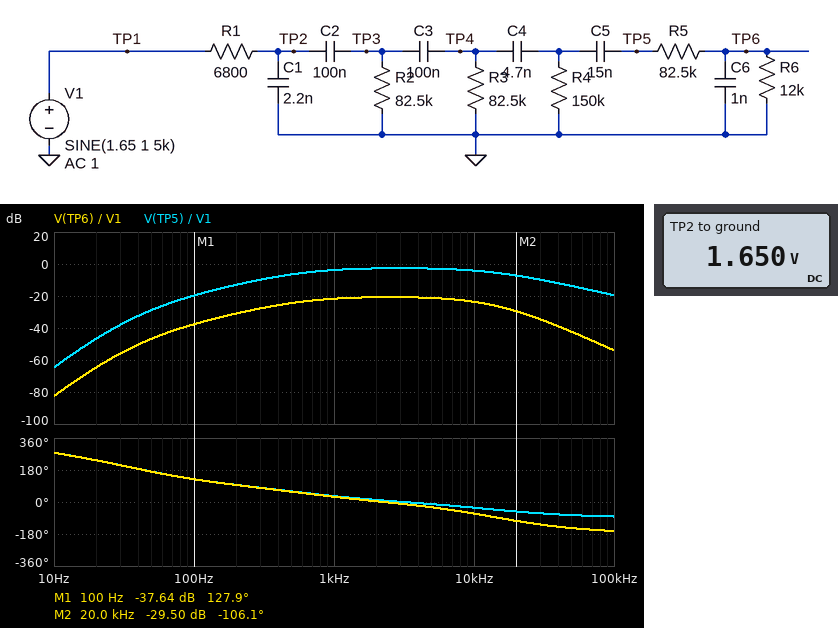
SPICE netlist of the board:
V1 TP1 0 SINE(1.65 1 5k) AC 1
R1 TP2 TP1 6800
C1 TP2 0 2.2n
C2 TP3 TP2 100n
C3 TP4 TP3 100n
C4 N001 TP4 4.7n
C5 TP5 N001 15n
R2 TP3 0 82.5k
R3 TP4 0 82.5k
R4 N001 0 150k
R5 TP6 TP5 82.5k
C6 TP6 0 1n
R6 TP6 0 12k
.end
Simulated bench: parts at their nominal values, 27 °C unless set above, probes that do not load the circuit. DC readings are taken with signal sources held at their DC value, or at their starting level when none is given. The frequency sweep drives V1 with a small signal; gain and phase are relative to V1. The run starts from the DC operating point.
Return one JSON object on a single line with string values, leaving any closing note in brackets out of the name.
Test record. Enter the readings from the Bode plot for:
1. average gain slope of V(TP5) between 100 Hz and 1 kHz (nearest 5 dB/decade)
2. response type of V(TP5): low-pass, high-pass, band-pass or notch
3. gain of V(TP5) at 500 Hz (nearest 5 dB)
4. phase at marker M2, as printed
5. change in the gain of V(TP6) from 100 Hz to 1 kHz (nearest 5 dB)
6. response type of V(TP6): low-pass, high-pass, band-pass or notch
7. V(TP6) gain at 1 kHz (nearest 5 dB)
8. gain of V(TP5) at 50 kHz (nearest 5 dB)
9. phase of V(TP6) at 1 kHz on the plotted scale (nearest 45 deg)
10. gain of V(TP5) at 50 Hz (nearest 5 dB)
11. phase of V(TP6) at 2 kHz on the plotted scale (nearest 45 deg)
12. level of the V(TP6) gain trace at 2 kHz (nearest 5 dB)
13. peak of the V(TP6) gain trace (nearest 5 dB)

{"average gain slope of V(TP5) between 100 Hz and 1 kHz": "15 dB/decade", "response type of V(TP5): low-pass, high-pass, band-pass or notch": "band-pass", "gain of V(TP5) at 500 Hz": "-5 dB", "phase at marker M2, as printed": "-106.1 deg", "change in the gain of V(TP6) from 100 Hz to 1 kHz": "15 dB", "response type of V(TP6): low-pass, high-pass, band-pass or notch": "band-pass", "V(TP6) gain at 1 kHz": "-20 dB", "gain of V(TP5) at 50 kHz": "-15 dB", "phase of V(TP6) at 1 kHz on the plotted scale": "45 deg", "gain of V(TP5) at 50 Hz": "-30 dB", "phase of V(TP6) at 2 kHz on the plotted scale": "0 deg", "level of the V(TP6) gain trace at 2 kHz": "-20 dB", "peak of the V(TP6) gain trace": "-20 dB"}
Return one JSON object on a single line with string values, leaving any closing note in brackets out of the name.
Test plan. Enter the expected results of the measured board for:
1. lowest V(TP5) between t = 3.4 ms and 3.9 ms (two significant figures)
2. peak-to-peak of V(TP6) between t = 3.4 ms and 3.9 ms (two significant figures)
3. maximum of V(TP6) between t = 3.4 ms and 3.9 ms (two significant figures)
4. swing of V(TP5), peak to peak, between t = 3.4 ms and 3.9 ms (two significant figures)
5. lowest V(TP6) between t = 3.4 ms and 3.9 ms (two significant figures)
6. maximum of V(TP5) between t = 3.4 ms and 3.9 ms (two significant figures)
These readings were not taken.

{"lowest V(TP5) between t = 3.4 ms and 3.9 ms": "-720 mV", "peak-to-peak of V(TP6) between t = 3.4 ms and 3.9 ms": "170 mV", "maximum of V(TP6) between t = 3.4 ms and 3.9 ms": "87 mV", "swing of V(TP5), peak to peak, between t = 3.4 ms and 3.9 ms": "1.4 V", "lowest V(TP6) between t = 3.4 ms and 3.9 ms": "-87 mV", "maximum of V(TP5) between t = 3.4 ms and 3.9 ms": "720 mV"}
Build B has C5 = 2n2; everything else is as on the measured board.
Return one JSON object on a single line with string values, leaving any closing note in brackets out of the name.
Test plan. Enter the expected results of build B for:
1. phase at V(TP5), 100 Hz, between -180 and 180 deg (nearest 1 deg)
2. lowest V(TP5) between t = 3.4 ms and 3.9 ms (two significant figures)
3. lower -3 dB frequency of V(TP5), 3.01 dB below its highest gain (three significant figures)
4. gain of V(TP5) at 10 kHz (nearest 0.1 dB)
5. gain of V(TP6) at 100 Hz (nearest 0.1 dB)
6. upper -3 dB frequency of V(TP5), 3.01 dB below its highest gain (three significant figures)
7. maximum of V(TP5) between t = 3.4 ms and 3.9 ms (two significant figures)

{"phase at V(TP5), 100 Hz, between -180 and 180 deg": "167 deg", "lowest V(TP5) between t = 3.4 ms and 3.9 ms": "-700 mV", "lower -3 dB frequency of V(TP5), 3.01 dB below its highest gain": "996 Hz", "gain of V(TP5) at 10 kHz": "-4.2 dB", "gain of V(TP6) at 100 Hz": "-47.1 dB", "upper -3 dB frequency of V(TP5), 3.01 dB below its highest gain": "15.9 kHz", "maximum of V(TP5) between t = 3.4 ms and 3.9 ms": "700 mV"}
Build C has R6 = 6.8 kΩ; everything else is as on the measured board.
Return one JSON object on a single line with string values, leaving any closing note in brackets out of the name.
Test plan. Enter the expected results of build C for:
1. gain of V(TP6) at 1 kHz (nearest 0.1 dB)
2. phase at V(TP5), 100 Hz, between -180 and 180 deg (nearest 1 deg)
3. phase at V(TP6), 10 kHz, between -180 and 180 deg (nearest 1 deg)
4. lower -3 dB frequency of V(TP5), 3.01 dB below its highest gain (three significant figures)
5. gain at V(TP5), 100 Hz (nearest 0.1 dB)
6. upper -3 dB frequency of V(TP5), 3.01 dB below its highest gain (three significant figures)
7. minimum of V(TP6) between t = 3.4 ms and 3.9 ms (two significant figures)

{"gain of V(TP6) at 1 kHz": "-26.2 dB", "phase at V(TP5), 100 Hz, between -180 and 180 deg": "129 deg", "phase at V(TP6), 10 kHz, between -180 and 180 deg": "-53 deg", "lower -3 dB frequency of V(TP5), 3.01 dB below its highest gain": "608 Hz", "gain at V(TP5), 100 Hz": "-20.1 dB", "upper -3 dB frequency of V(TP5), 3.01 dB below its highest gain": "15.0 kHz", "minimum of V(TP6) between t = 3.4 ms and 3.9 ms": "-54 mV"}
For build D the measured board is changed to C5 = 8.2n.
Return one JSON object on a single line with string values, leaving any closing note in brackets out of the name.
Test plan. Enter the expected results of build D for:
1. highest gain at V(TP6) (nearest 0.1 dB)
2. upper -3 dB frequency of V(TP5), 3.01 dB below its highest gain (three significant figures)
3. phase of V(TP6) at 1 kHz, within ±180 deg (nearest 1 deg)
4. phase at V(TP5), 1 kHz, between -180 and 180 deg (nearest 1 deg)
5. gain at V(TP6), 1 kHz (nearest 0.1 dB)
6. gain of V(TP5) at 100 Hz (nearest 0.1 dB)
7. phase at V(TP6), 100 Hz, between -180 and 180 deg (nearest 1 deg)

{"highest gain at V(TP6)": "-20.8 dB", "upper -3 dB frequency of V(TP5), 3.01 dB below its highest gain": "15.0 kHz", "phase of V(TP6) at 1 kHz, within ±180 deg": "33 deg", "phase at V(TP5), 1 kHz, between -180 and 180 deg": "37 deg", "gain at V(TP6), 1 kHz": "-22.0 dB", "gain of V(TP5) at 100 Hz": "-21.4 dB", "phase at V(TP6), 100 Hz, between -180 and 180 deg": "140 deg"}
